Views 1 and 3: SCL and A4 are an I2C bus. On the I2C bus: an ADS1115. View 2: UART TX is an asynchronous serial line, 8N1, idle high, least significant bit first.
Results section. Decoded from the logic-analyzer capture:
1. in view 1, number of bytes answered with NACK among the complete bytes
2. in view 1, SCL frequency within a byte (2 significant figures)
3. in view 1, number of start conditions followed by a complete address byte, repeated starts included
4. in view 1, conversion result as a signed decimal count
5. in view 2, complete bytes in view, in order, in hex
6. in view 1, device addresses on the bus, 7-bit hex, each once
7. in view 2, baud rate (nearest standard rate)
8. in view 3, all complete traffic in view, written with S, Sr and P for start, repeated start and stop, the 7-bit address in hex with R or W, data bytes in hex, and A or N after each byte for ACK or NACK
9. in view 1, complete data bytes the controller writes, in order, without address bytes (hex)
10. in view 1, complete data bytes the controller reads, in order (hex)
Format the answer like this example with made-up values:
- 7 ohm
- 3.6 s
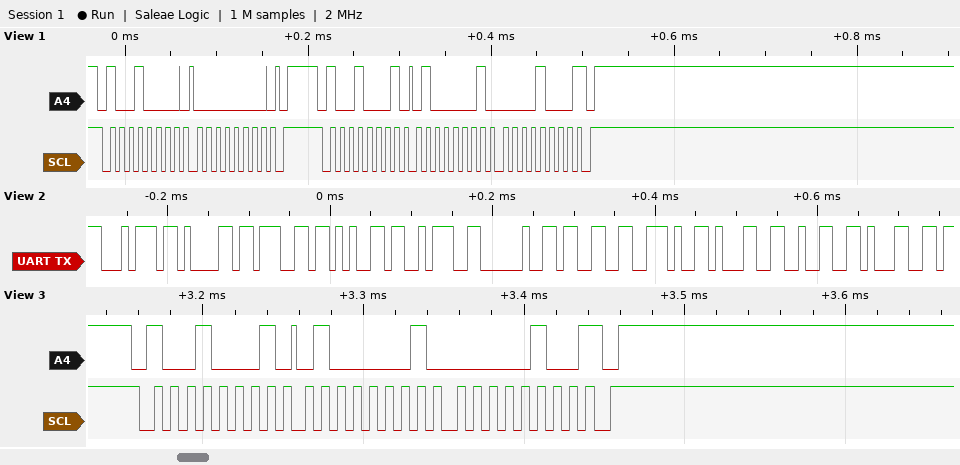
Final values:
- 1
- 100 kHz
- 2
- 16648
- 74 61 67 65 3A 20 33 2E 31 32 31
- 0x48
- 115200 baud
- S 48R A 41 A 04 N P
- 00
- 41 08
